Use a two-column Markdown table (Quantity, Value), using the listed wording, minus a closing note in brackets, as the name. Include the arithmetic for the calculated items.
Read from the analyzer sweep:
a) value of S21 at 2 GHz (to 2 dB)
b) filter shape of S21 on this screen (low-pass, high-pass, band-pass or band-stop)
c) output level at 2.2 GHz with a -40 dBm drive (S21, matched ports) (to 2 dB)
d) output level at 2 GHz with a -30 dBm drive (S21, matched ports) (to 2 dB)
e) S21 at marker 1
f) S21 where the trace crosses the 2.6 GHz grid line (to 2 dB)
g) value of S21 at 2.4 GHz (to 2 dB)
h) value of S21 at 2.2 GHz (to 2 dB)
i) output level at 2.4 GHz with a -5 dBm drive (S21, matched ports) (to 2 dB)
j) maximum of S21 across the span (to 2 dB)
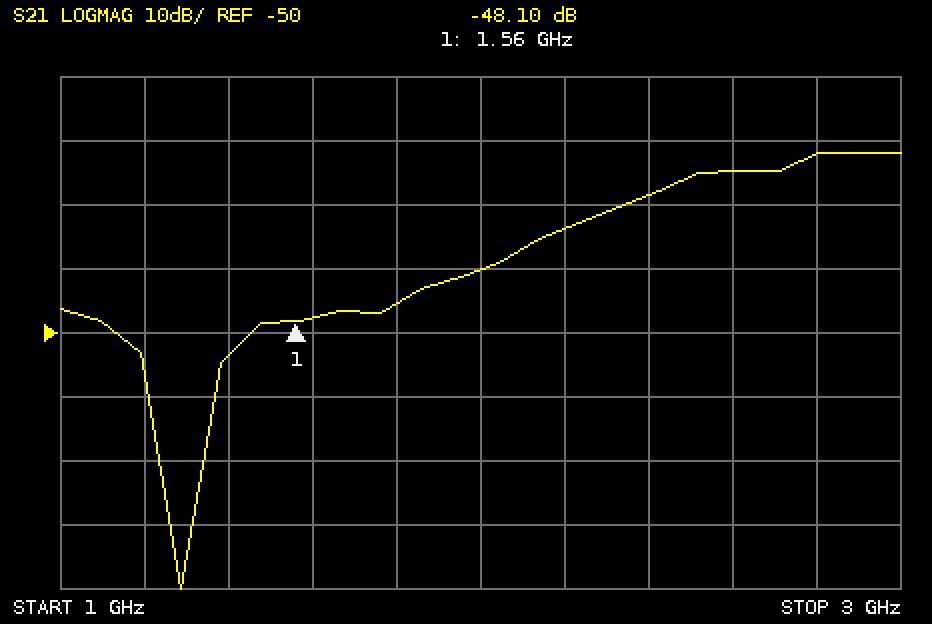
| Quantity | Value |
|---|---|
| value of S21 at 2 GHz | -40 dB |
| filter shape of S21 on this screen | high-pass |
| output level at 2.2 GHz with a -40 dBm drive (S21, matched ports) | -40 dBm + (-34 dB) = -74 dBm |
| output level at 2 GHz with a -30 dBm drive (S21, matched ports) | -30 dBm + (-40 dB) = -70 dBm |
| S21 at marker 1 | -48.10 dB |
| S21 where the trace crosses the 2.6 GHz grid line | -24 dB |
| value of S21 at 2.4 GHz | -28 dB |
| value of S21 at 2.2 GHz | -34 dB |
| output level at 2.4 GHz with a -5 dBm drive (S21, matched ports) | -5 dBm + (-28 dB) = -34 dBm |
| maximum of S21 across the span | -22 dB |
